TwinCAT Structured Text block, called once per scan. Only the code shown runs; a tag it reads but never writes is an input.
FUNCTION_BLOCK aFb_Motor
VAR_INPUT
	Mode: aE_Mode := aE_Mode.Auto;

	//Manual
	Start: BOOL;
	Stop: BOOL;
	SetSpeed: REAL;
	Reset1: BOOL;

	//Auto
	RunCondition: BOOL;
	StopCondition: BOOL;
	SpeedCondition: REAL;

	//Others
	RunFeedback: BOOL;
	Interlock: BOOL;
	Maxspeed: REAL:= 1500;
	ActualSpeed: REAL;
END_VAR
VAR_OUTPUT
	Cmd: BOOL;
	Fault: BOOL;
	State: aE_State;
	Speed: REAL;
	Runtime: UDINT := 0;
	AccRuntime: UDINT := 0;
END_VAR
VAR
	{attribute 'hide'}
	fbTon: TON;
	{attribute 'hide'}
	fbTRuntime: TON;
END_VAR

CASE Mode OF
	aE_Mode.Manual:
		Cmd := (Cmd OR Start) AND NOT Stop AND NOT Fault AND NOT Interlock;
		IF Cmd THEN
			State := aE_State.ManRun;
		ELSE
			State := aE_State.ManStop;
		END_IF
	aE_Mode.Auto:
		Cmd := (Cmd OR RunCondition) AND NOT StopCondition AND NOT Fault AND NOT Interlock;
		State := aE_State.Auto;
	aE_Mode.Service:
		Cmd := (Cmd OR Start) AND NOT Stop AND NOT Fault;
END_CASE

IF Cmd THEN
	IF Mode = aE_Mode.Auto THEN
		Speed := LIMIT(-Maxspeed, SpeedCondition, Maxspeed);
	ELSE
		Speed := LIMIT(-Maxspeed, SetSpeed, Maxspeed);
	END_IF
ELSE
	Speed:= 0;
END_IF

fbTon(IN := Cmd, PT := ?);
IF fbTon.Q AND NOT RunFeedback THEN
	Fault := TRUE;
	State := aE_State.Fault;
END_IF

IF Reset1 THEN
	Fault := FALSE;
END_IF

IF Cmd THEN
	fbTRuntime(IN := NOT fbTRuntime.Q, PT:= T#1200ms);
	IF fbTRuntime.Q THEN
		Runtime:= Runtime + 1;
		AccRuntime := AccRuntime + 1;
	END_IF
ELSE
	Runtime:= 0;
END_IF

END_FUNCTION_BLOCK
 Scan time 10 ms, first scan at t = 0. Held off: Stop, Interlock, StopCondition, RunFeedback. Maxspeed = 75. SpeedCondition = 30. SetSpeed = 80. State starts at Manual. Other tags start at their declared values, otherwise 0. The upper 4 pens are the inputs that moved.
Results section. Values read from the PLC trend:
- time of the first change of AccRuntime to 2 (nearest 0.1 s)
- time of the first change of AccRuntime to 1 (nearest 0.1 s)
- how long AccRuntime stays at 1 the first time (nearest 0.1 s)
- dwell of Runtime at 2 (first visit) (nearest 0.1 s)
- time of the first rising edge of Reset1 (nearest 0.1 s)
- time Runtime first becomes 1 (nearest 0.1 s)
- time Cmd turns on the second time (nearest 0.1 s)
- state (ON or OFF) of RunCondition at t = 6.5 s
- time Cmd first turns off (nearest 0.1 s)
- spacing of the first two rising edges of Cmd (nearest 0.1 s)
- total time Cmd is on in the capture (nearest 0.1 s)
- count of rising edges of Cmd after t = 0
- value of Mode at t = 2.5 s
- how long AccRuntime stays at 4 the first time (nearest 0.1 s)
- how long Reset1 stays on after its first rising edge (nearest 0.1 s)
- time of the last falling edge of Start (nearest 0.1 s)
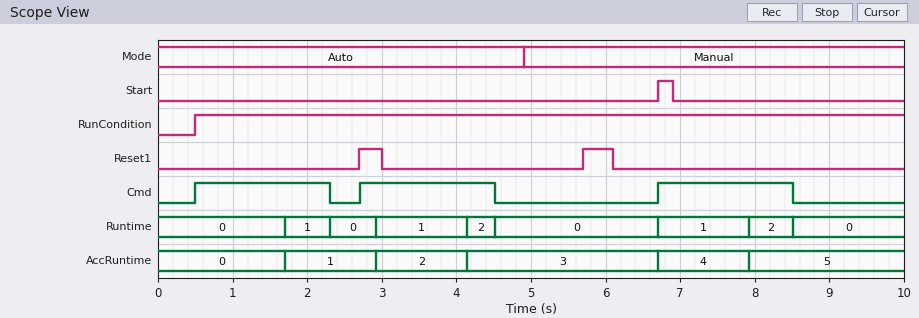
2.9 s
1.7 s
1.2 s
0.4 s
2.7 s
1.7 s
2.7 s
ON
2.3 s
2.2 s
5.4 s
3
Auto
1.2 s
0.3 s
6.9 s
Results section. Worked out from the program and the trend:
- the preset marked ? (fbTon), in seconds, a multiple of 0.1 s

1.8 s
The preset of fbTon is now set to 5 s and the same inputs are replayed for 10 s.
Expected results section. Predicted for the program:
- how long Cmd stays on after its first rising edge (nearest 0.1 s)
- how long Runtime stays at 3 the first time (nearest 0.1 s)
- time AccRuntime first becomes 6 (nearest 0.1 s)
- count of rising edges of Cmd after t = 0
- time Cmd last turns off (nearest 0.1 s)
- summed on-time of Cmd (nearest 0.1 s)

5.0 s
1.2 s
7.9 s
2
5.5 s
8.3 s
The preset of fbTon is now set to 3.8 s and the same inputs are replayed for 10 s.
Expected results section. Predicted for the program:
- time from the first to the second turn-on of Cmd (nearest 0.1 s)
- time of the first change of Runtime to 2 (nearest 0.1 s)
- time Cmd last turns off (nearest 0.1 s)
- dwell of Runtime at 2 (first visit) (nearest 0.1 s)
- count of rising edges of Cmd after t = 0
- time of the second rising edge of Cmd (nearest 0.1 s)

6.2 s
2.9 s
4.3 s
1.2 s
2
6.7 s
